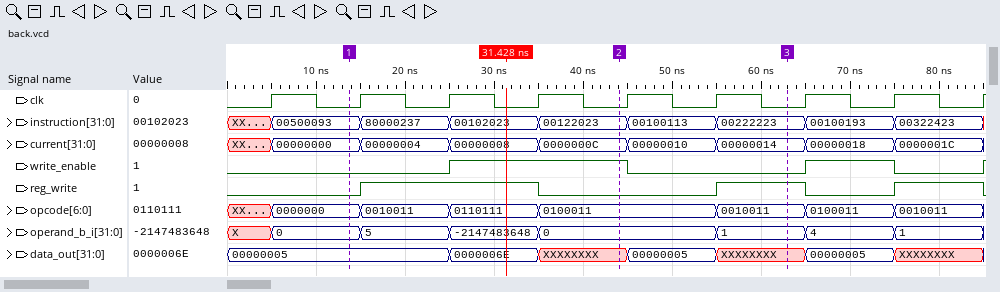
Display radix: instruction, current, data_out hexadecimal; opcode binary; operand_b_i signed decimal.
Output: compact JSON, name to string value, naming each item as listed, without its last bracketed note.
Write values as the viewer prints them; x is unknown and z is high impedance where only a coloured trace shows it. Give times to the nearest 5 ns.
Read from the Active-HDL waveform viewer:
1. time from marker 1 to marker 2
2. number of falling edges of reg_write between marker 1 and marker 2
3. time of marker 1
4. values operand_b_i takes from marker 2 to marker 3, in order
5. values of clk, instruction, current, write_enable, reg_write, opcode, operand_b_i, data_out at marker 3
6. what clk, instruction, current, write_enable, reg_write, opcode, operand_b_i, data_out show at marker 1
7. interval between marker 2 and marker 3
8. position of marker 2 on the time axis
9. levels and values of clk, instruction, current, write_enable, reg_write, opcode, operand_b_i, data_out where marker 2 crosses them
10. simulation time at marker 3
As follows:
{"time from marker 1 to marker 2": "30 ns", "number of falling edges of reg_write between marker 1 and marker 2": "1", "time of marker 1": "15 ns", "values operand_b_i takes from marker 2 to marker 3, in order": "0, 1", "values of clk, instruction, current, write_enable, reg_write, opcode, operand_b_i, data_out at marker 3": "clk=0, instruction=00222223, current=00000014, write_enable=0, reg_write=1, opcode=0010011, operand_b_i=1, data_out=XXXXXXXX", "what clk, instruction, current, write_enable, reg_write, opcode, operand_b_i, data_out show at marker 1": "clk=0, instruction=00500093, current=00000000, write_enable=0, reg_write=0, opcode=0000000, operand_b_i=0, data_out=00000005", "interval between marker 2 and marker 3": "20 ns", "position of marker 2 on the time axis": "45 ns", "levels and values of clk, instruction, current, write_enable, reg_write, opcode, operand_b_i, data_out where marker 2 crosses them": "clk=0, instruction=00122023, current=0000000C, write_enable=1, reg_write=0, opcode=0100011, operand_b_i=0, data_out=XXXXXXXX", "simulation time at marker 3": "65 ns"}
